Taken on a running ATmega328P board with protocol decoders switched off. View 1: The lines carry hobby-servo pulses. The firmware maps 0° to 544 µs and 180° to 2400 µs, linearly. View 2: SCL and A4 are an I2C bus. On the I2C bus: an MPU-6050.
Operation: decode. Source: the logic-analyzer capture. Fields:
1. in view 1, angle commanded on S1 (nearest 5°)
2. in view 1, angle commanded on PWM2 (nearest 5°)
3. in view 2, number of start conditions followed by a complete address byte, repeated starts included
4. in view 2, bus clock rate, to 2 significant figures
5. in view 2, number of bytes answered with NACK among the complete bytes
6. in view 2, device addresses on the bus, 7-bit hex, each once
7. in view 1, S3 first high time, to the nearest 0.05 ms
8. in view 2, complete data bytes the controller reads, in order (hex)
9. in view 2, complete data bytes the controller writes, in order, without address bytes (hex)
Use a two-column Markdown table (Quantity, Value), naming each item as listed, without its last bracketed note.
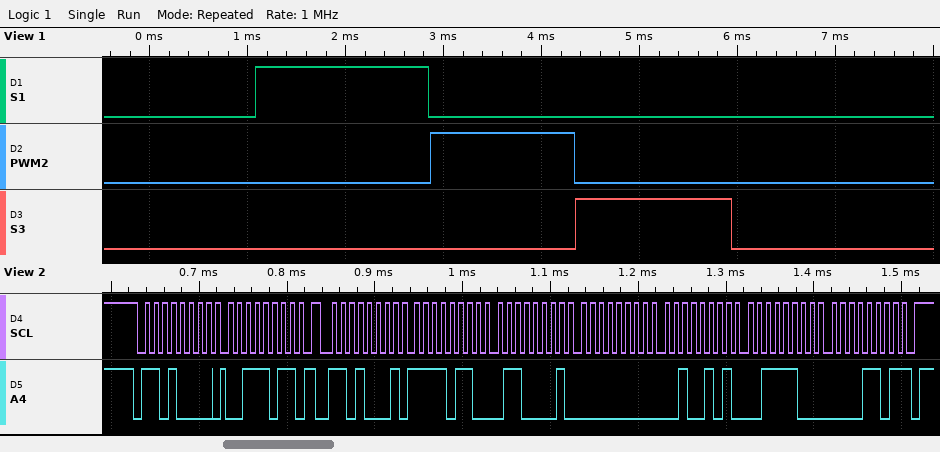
| Quantity | Value |
|---|---|
| in view 1, angle commanded on S1 | 120° |
| in view 1, angle commanded on PWM2 | 90° |
| in view 2, number of start conditions followed by a complete address byte, repeated starts included | 2 |
| in view 2, bus clock rate, to 2 significant figures | 100 kHz |
| in view 2, number of bytes answered with NACK among the complete bytes | 1 |
| in view 2, device addresses on the bus, 7-bit hex, each once | 0x68 |
| in view 1, S3 first high time, to the nearest 0.05 ms | 1.60 ms |
| in view 2, complete data bytes the controller reads, in order | F6 61 00 25 3C 0D |
| in view 2, complete data bytes the controller writes, in order, without address bytes | 3B |
